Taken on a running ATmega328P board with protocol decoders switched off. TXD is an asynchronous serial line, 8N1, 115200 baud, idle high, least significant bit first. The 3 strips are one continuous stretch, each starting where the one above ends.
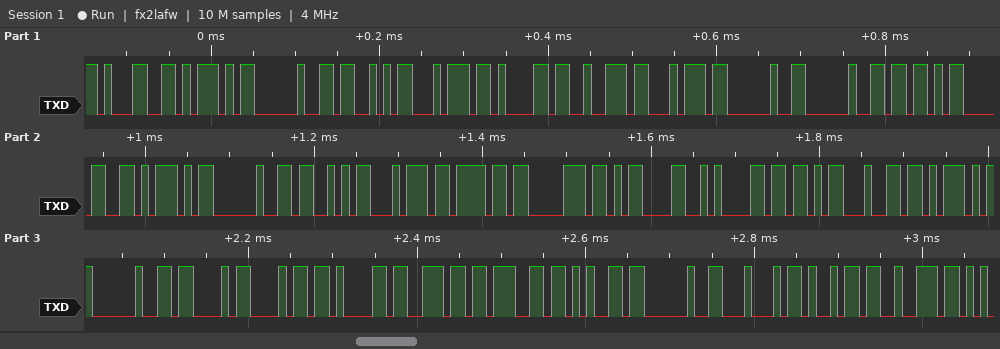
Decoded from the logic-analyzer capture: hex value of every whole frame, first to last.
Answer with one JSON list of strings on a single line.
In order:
["31 5D 20 53 74 61 72 74 20 20 5B 30 5D 20 53 74 6F 70 0D 0A 5B 64 5D 20 43 68 61 6E 67 65 20 44 69 72"]
